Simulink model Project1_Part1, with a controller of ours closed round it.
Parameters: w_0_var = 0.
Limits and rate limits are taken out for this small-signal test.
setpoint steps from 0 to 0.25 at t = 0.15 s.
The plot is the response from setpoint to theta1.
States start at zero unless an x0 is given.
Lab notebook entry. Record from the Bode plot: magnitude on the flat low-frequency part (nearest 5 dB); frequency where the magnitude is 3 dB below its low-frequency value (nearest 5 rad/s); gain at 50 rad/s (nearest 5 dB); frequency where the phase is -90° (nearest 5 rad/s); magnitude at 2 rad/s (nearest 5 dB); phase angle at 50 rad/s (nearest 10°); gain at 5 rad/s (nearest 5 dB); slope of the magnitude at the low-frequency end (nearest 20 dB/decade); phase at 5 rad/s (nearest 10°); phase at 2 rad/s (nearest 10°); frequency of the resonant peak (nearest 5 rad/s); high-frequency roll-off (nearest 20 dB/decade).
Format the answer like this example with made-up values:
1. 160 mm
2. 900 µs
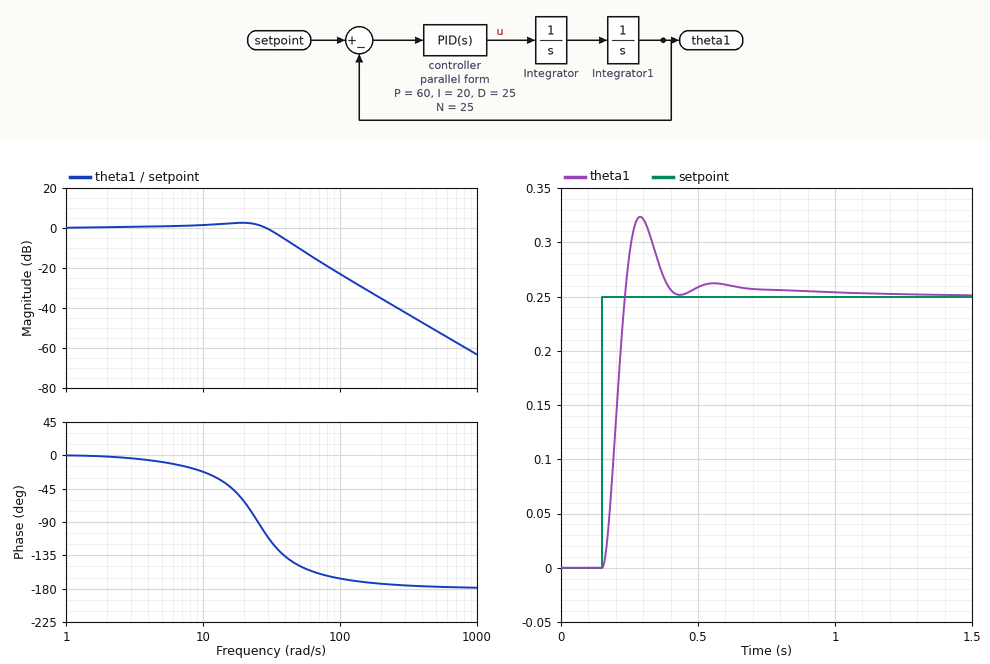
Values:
1. 0 dB
2. 35 rad/s
3. -10 dB
4. 25 rad/s
5. 0 dB
6. -150°
7. 0 dB
8. 0 dB/decade
9. -10°
10. 0°
11. 20 rad/s
12. -40 dB/decade
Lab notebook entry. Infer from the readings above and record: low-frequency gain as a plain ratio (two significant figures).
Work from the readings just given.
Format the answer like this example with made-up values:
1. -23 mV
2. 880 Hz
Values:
1. 1.0
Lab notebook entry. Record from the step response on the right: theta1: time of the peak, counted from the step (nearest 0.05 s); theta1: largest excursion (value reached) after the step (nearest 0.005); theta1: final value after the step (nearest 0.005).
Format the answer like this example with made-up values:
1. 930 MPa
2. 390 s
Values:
1. 0.15 s
2. 0.325
3. 0.250
